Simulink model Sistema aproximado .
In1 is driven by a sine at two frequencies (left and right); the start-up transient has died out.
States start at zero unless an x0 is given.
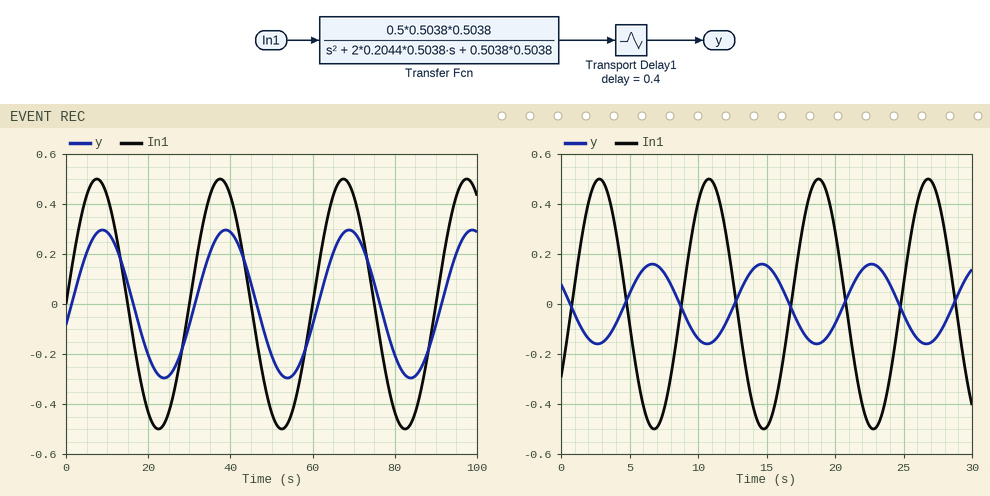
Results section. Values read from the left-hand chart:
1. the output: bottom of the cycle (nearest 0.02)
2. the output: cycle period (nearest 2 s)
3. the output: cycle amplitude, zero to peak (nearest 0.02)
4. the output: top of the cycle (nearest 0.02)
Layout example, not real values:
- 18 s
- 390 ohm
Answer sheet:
- -0.30
- 30 s
- 0.30
- 0.30
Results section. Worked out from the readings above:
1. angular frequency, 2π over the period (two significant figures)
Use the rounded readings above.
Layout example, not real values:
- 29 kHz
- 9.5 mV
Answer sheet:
- 0.21 rad/s
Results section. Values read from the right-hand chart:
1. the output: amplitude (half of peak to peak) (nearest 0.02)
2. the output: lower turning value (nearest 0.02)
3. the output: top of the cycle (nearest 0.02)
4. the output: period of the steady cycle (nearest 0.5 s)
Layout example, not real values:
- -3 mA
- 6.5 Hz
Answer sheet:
- 0.16
- -0.16
- 0.16
- 8.0 s
